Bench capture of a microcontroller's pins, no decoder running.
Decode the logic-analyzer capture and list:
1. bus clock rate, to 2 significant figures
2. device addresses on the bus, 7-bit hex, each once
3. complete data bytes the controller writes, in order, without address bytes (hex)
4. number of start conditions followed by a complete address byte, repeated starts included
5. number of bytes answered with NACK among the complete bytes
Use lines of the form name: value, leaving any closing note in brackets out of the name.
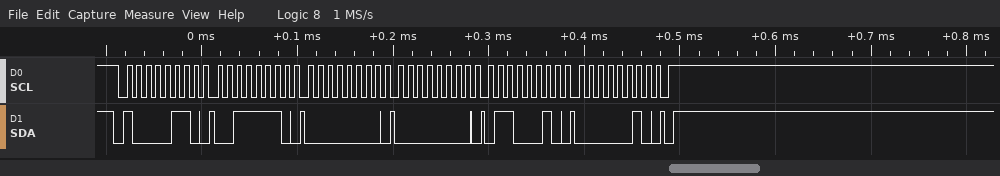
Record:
bus clock rate, to 2 significant figures: 100 kHz
device addresses on the bus, 7-bit hex, each once: 0x43
complete data bytes the controller writes, in order, without address bytes: 3E 00 00 62 02
number of start conditions followed by a complete address byte, repeated starts included: 1
number of bytes answered with NACK among the complete bytes: 0
